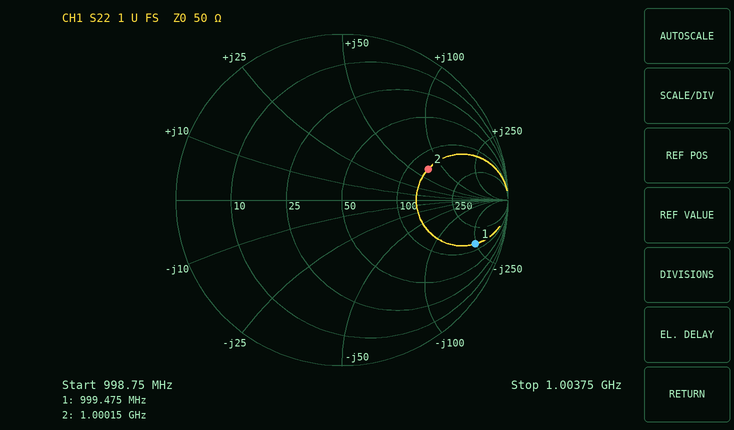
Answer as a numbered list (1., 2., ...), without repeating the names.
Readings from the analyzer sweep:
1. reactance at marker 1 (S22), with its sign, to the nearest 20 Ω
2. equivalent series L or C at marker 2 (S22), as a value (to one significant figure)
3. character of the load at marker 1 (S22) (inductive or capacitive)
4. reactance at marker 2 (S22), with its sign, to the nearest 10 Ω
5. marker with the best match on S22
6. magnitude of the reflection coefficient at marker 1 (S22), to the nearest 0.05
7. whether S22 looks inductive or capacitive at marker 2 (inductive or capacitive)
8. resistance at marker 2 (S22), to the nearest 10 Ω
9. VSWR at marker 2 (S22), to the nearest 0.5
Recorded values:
1. -240 Ω
2. 10 nH
3. capacitive
4. +70 Ω
5. marker 2
6. 0.85
7. inductive
8. 130 Ω
9. 3.5
